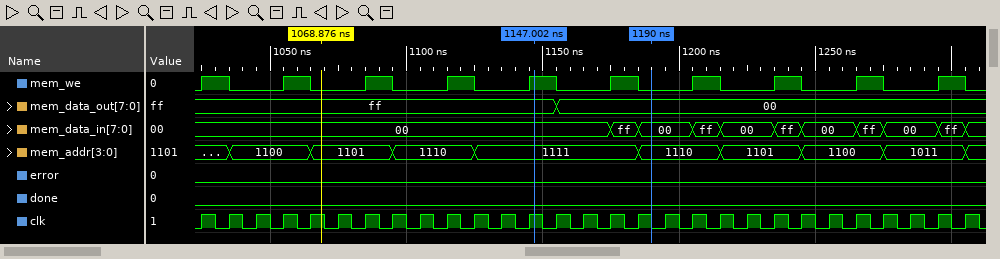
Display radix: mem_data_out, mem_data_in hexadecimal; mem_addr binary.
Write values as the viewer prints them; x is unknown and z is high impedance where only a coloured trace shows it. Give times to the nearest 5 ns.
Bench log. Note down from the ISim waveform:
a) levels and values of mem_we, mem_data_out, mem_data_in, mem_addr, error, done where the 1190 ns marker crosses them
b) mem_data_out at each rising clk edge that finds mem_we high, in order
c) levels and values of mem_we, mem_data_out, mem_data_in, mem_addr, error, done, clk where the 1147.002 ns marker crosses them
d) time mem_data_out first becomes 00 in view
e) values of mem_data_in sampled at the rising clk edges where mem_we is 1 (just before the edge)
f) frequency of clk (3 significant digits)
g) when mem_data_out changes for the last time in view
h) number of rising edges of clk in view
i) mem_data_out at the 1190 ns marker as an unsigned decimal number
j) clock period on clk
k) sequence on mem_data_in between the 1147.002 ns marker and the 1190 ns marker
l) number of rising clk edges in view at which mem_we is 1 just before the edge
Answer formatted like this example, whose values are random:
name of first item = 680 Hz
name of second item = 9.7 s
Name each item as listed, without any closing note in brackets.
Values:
levels and values of mem_we, mem_data_out, mem_data_in, mem_addr, error, done where the 1190 ns marker crosses them = mem_we=0, mem_data_out=00, mem_data_in=00, mem_addr=1110, error=0, done=0
mem_data_out at each rising clk edge that finds mem_we high, in order = ff, ff, ff, ff, ff, 00, 00, 00, 00, 00
levels and values of mem_we, mem_data_out, mem_data_in, mem_addr, error, done, clk where the 1147.002 ns marker crosses them = mem_we=1, mem_data_out=ff, mem_data_in=00, mem_addr=1111, error=0, done=0, clk=1
time mem_data_out first becomes 00 in view = 1155 ns
values of mem_data_in sampled at the rising clk edges where mem_we is 1 = 00, 00, 00, 00, 00, ff, ff, ff, ff, ff
frequency of clk = 100 MHz
when mem_data_out changes for the last time in view = 1155 ns
number of rising edges of clk in view = 29
mem_data_out at the 1190 ns marker as an unsigned decimal number = 0
clock period on clk = 10 ns
sequence on mem_data_in between the 1147.002 ns marker and the 1190 ns marker = 00, ff, 00
number of rising clk edges in view at which mem_we is 1 just before the edge = 10
